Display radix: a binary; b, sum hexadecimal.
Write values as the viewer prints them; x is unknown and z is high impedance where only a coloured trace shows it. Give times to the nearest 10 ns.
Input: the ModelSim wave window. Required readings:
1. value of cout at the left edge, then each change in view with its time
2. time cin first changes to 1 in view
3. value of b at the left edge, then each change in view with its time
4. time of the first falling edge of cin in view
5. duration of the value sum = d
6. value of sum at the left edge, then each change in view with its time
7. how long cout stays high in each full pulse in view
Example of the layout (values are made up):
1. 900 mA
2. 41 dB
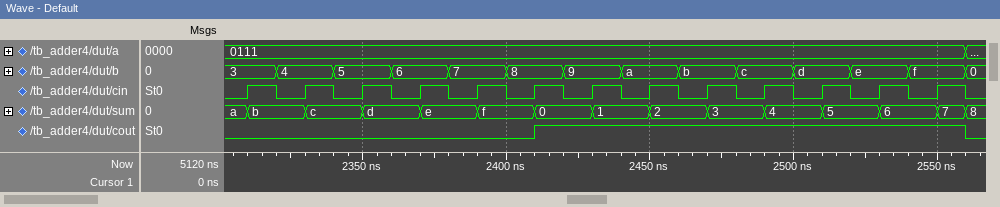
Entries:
1. 0, 1 at 2410 ns, 0 at 2560 ns
2. 2310 ns
3. 3, 4 at 2320 ns, 5 at 2340 ns, 6 at 2360 ns, 7 at 2380 ns, 8 at 2400 ns, 9 at 2420 ns, a at 2440 ns, b at 2460 ns, c at 2480 ns, d at 2500 ns, e at 2520 ns, f at 2540 ns, 0 at 2560 ns
4. 2320 ns
5. 20 ns
6. a, b at 2310 ns, c at 2330 ns, d at 2350 ns, e at 2370 ns, f at 2390 ns, 0 at 2410 ns, 1 at 2430 ns, 2 at 2450 ns, 3 at 2470 ns, 4 at 2490 ns, 5 at 2510 ns, 6 at 2530 ns, 7 at 2550 ns, 8 at 2560 ns
7. 150 ns
